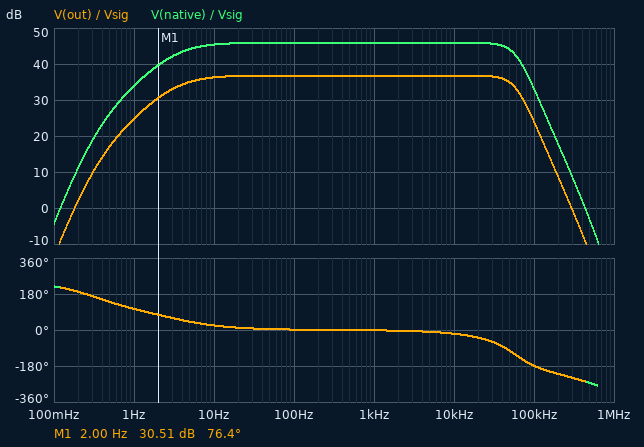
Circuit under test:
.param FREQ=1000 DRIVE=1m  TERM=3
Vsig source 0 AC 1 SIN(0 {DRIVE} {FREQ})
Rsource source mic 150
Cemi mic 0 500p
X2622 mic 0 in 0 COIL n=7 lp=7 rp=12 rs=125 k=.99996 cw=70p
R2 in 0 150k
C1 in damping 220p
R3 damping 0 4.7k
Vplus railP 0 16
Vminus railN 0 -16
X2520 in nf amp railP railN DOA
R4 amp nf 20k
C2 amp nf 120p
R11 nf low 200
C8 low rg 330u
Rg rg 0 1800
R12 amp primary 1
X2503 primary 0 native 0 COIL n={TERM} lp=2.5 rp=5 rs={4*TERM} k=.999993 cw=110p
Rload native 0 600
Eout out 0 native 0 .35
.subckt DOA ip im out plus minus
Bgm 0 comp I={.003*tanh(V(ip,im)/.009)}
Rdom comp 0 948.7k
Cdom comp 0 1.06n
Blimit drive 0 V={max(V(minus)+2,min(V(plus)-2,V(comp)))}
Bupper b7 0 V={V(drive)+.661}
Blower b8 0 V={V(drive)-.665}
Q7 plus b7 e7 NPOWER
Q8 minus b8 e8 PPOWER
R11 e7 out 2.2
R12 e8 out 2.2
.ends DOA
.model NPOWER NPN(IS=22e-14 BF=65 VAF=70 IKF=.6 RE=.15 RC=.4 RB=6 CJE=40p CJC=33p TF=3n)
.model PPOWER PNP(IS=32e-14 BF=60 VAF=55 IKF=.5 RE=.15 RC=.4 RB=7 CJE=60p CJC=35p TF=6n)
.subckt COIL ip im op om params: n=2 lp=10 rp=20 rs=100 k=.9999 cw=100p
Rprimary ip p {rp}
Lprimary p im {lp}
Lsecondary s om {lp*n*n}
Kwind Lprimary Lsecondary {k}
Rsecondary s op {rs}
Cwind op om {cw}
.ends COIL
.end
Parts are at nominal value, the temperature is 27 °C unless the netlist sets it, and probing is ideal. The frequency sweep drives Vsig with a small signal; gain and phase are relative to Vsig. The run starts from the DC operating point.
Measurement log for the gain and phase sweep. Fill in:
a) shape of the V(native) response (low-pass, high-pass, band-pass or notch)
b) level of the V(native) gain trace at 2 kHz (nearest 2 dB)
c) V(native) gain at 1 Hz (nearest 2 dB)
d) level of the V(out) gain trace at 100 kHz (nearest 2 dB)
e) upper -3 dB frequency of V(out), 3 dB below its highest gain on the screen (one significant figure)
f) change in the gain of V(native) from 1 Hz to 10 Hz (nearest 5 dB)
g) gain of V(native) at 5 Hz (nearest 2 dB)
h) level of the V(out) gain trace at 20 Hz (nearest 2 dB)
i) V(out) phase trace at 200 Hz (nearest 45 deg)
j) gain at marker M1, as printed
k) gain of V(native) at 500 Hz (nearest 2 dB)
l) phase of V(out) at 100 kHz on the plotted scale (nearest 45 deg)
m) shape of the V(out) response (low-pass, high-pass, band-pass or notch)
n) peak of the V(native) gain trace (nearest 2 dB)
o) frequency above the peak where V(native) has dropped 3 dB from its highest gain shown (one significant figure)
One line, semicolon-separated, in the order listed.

band-pass; 46 dB; 34 dB; 24 dB; 60 kHz; 10 dB; 44 dB; 36 dB; 0 deg; 30.51 dB; 46 dB; -180 deg; band-pass; 46 dB; 60 kHz
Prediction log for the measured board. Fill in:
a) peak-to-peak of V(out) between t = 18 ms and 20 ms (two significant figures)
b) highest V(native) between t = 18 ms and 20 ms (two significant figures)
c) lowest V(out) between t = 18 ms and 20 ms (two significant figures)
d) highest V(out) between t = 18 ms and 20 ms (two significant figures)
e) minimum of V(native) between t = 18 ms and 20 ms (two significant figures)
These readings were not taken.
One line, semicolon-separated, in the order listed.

140 mV; 200 mV; -69 mV; 69 mV; -200 mV
